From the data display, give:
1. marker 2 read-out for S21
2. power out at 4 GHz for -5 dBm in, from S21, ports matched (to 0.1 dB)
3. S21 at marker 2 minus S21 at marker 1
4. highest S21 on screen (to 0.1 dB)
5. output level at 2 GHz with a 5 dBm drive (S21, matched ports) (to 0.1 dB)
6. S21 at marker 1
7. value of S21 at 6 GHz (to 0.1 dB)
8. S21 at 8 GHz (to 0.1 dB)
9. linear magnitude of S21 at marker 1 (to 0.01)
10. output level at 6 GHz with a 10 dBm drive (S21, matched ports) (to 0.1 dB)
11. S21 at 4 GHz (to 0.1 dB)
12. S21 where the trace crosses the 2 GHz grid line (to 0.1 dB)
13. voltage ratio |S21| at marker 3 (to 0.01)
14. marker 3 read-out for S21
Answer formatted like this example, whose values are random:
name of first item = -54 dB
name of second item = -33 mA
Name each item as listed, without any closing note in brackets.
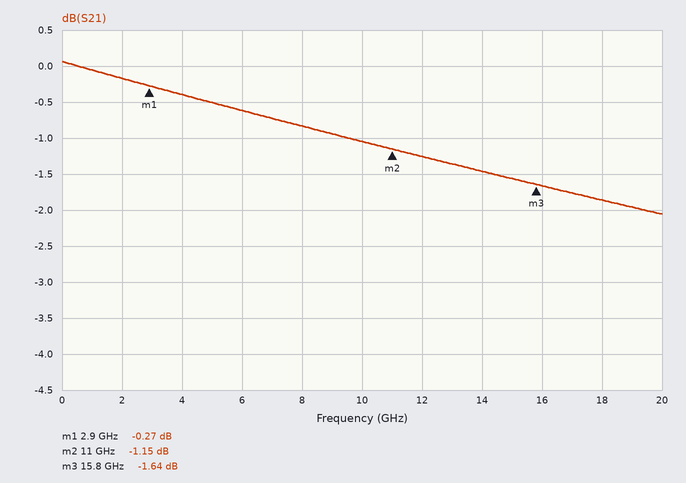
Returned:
marker 2 read-out for S21 = -1.15 dB
power out at 4 GHz for -5 dBm in, from S21, ports matched = -5.4 dBm
S21 at marker 2 minus S21 at marker 1 = -0.88 dB
highest S21 on screen = 0.1 dB
output level at 2 GHz with a 5 dBm drive (S21, matched ports) = 4.8 dBm
S21 at marker 1 = -0.27 dB
value of S21 at 6 GHz = -0.6 dB
S21 at 8 GHz = -0.8 dB
linear magnitude of S21 at marker 1 = 0.97
output level at 6 GHz with a 10 dBm drive (S21, matched ports) = 9.4 dBm
S21 at 4 GHz = -0.4 dB
S21 where the trace crosses the 2 GHz grid line = -0.2 dB
voltage ratio |S21| at marker 3 = 0.83
marker 3 read-out for S21 = -1.64 dB
